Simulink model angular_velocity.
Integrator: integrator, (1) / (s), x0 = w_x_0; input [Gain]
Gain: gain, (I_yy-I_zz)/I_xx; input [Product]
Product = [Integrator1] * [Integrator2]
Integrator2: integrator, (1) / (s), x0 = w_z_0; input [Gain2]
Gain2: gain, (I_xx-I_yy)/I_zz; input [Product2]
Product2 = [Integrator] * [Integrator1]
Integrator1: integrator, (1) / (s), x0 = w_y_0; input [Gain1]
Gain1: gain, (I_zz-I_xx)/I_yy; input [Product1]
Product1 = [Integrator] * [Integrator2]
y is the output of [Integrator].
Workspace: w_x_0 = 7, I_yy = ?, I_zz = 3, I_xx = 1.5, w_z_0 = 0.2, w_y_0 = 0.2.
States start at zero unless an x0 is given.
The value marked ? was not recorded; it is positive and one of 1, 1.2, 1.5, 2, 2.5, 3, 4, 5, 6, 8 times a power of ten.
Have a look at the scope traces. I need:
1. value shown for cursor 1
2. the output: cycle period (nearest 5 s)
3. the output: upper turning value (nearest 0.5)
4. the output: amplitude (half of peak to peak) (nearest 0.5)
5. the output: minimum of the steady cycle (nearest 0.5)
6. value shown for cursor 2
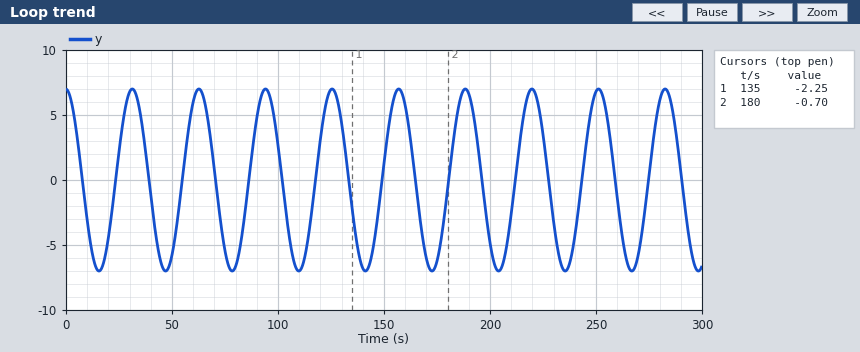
-2.25
30 s
7.0
7.0
-7.0
-0.70
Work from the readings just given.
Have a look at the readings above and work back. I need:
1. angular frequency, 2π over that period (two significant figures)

0.21 rad/s
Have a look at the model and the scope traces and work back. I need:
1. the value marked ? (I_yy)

1.5
